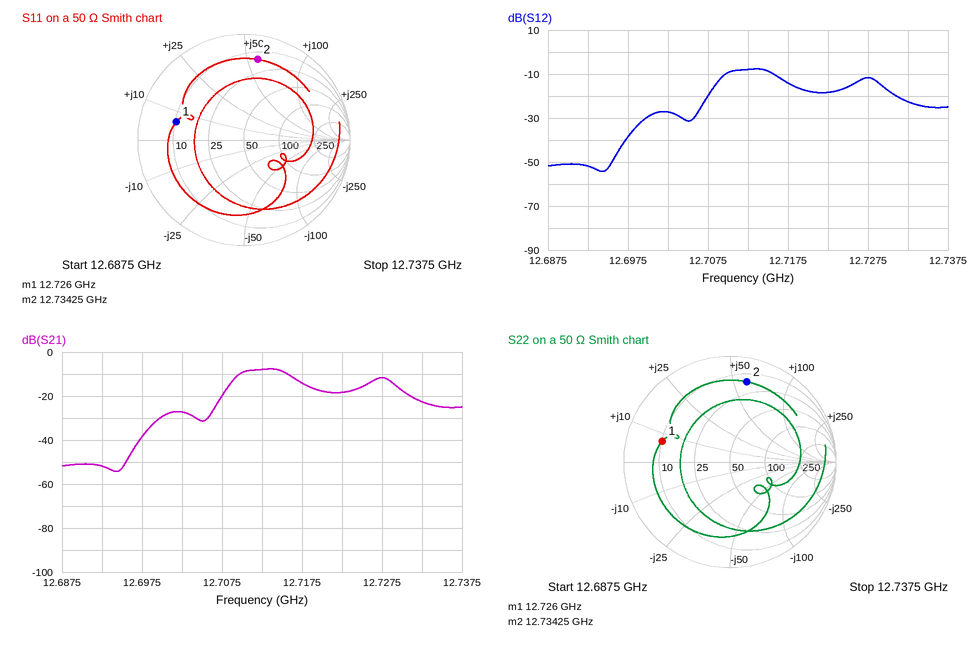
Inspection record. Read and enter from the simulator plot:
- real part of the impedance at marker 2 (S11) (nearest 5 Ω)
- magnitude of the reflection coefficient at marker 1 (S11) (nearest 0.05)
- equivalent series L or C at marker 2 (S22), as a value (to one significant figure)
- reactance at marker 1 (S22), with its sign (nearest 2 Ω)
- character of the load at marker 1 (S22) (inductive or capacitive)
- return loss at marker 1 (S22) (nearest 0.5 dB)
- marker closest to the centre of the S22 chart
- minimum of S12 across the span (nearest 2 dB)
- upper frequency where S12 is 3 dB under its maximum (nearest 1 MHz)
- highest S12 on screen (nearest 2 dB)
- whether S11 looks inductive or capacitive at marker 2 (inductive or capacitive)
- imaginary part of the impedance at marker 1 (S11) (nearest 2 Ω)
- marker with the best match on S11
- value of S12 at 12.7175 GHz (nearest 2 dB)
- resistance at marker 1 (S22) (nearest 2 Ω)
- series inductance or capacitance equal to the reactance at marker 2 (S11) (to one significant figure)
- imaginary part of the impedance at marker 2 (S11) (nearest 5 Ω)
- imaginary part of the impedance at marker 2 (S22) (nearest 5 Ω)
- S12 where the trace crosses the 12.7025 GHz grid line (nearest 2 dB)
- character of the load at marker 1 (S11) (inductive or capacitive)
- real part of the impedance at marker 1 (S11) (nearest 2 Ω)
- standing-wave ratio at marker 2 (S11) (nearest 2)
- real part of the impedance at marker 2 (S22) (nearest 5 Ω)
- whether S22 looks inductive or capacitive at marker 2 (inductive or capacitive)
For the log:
15 Ω
0.65
700 pH
+8 Ω
inductive
3.5 dB
marker 1
-54 dB
12.716 GHz
-8 dB
inductive
+6 Ω
marker 1
-14 dB
10 Ω
700 pH
+55 Ω
+60 Ω
-28 dB
inductive
10 Ω
8
15 Ω
inductive
